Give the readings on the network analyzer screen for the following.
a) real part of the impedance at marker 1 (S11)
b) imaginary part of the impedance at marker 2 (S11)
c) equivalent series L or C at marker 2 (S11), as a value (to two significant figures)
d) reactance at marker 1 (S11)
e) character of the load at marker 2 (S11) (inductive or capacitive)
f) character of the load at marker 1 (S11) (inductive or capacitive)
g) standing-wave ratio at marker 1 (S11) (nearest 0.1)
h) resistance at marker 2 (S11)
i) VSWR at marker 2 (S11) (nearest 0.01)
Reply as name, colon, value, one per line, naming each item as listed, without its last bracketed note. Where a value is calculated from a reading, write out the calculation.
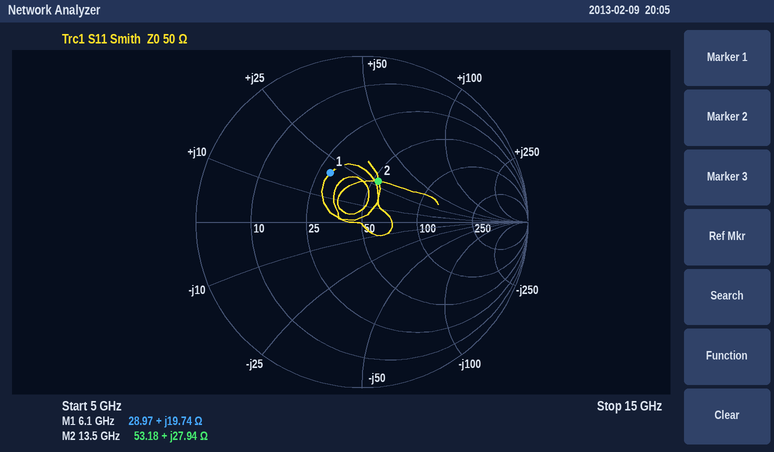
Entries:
real part of the impedance at marker 1: 28.97 Ω
imaginary part of the impedance at marker 2: +27.94 Ω
equivalent series L or C at marker 2 (S11), as a value: L = 27.94 Ω/(2π × 13.5 GHz) ≈ 329 pH, so 330 pH to two significant figures
reactance at marker 1: +19.74 Ω
character of the load at marker 2 (S11): inductive
character of the load at marker 1 (S11): inductive
standing-wave ratio at marker 1 (S11): 2.1
resistance at marker 2: 53.18 Ω
VSWR at marker 2 (S11): 1.71
